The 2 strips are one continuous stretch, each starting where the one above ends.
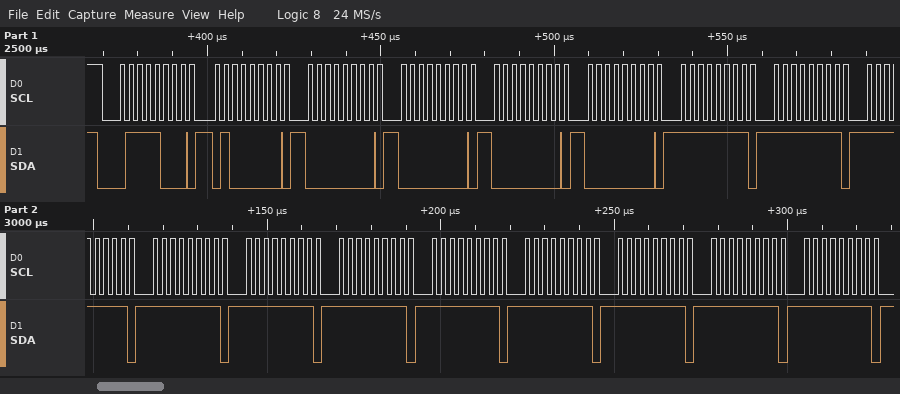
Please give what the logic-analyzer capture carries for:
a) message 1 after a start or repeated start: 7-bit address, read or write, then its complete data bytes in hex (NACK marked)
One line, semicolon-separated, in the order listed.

0x3C write: 40 00 00 00 00 FF FF FF FF FF FF FF FF FF FF FF
